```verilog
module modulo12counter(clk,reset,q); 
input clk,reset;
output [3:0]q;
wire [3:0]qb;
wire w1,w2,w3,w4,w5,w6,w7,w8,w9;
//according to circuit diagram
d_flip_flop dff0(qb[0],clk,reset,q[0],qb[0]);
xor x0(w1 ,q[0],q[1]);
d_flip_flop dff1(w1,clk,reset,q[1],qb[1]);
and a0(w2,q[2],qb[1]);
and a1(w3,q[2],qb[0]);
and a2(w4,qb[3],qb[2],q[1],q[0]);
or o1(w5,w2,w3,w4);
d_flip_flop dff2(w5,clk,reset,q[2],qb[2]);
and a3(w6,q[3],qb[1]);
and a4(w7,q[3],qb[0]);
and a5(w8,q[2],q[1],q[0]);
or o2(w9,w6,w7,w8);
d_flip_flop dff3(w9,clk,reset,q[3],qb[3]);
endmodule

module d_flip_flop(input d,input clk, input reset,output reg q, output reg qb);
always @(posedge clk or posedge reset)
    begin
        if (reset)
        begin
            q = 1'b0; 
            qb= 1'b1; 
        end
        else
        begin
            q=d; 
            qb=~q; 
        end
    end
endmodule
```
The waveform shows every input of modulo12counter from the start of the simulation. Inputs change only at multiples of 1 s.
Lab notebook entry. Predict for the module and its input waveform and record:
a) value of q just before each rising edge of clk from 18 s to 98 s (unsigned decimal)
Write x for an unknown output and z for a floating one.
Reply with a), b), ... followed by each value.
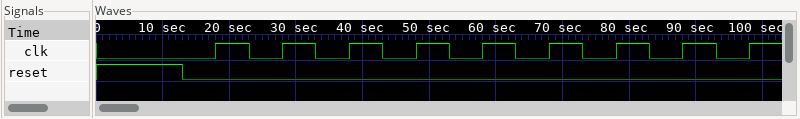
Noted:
a) 0, 1, 2, 3, 4, 5, 6, 7, 8
